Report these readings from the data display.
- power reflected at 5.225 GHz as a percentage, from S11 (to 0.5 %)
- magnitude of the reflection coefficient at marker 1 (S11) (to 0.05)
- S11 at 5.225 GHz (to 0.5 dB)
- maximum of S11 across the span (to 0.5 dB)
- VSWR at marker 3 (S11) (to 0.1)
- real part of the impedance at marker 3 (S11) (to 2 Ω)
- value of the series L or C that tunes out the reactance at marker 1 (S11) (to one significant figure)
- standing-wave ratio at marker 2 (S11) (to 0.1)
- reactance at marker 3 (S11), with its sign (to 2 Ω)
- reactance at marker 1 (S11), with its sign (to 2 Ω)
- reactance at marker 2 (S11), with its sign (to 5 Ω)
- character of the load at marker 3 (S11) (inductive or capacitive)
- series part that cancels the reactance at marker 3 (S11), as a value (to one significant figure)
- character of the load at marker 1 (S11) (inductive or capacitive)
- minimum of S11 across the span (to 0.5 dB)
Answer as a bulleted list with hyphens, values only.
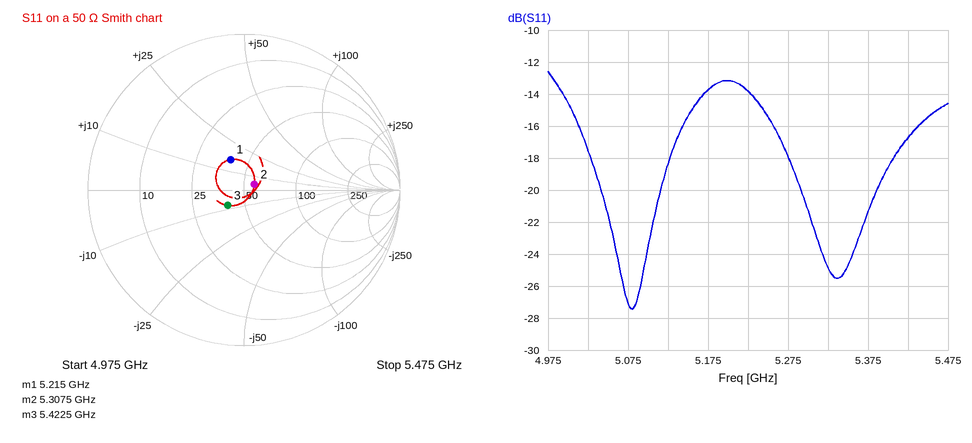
- 4.0 %
- 0.20
- -14.0 dB
- -12.5 dB
- 1.3
- 40 Ω
- 2 pF
- 1.2
- -8 Ω
- +16 Ω
- +5 Ω
- capacitive
- 200 pH
- inductive
- -27.5 dB
